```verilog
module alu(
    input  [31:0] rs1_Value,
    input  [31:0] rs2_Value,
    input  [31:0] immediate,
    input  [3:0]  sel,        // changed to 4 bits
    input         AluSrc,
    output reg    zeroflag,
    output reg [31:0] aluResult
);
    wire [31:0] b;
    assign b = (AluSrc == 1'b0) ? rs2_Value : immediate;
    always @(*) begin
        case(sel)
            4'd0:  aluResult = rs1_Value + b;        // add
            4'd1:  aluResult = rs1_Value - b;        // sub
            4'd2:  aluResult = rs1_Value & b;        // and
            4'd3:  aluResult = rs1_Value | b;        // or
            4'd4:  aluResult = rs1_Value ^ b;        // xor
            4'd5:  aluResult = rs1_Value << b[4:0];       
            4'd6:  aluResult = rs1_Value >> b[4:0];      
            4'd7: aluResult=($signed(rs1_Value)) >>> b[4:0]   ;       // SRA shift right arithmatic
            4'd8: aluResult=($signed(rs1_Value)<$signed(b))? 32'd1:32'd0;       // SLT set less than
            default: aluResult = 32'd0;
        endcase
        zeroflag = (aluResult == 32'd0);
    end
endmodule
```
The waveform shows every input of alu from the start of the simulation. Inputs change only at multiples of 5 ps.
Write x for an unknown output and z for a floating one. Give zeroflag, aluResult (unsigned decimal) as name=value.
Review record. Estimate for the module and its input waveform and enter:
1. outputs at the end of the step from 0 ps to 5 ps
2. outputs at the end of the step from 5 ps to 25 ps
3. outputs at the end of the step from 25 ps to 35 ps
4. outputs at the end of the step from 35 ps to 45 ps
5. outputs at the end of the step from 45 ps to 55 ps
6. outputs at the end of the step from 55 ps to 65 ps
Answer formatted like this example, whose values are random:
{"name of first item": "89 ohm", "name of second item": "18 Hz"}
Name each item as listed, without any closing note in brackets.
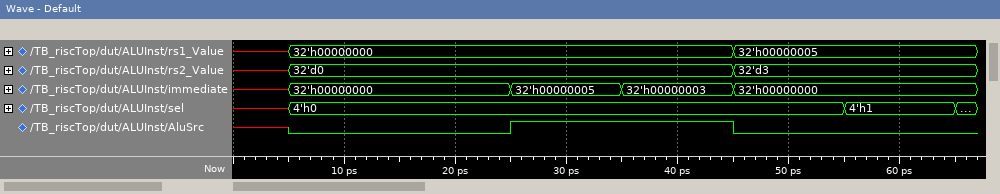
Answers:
{"outputs at the end of the step from 0 ps to 5 ps": "zeroflag=x, aluResult=x", "outputs at the end of the step from 5 ps to 25 ps": "zeroflag=1, aluResult=0", "outputs at the end of the step from 25 ps to 35 ps": "zeroflag=0, aluResult=5", "outputs at the end of the step from 35 ps to 45 ps": "zeroflag=0, aluResult=3", "outputs at the end of the step from 45 ps to 55 ps": "zeroflag=0, aluResult=8", "outputs at the end of the step from 55 ps to 65 ps": "zeroflag=0, aluResult=2"}
